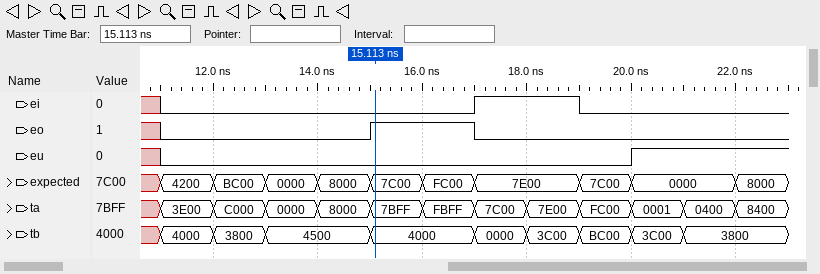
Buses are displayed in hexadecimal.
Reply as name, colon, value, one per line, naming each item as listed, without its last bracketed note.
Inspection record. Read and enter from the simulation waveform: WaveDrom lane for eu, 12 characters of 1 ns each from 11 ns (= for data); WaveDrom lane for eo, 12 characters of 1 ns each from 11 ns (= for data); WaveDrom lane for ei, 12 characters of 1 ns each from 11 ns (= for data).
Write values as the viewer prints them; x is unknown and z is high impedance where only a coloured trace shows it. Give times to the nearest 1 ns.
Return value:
WaveDrom lane for eu, 12 characters of 1 ns each from 11 ns: {name: 'eu', wave: '0........1..'}
WaveDrom lane for eo, 12 characters of 1 ns each from 11 ns: {name: 'eo', wave: '0...1.0.....'}
WaveDrom lane for ei, 12 characters of 1 ns each from 11 ns: {name: 'ei', wave: '0.....1.0...'}
